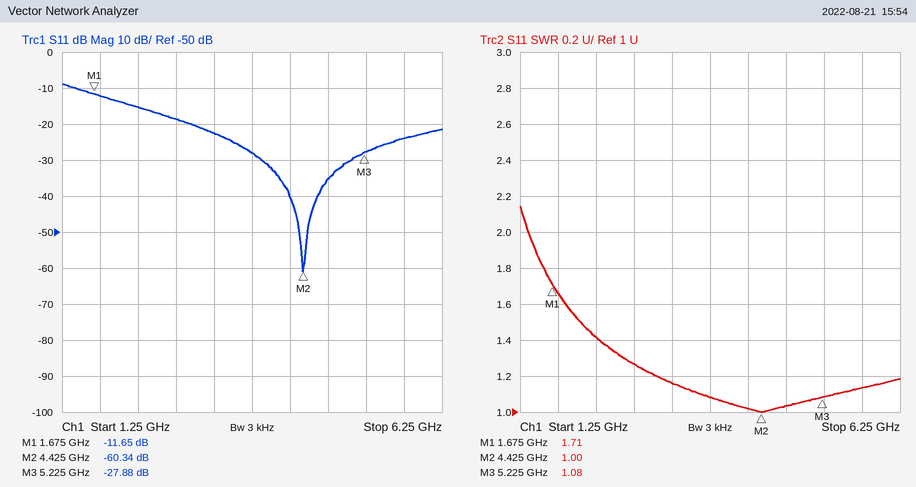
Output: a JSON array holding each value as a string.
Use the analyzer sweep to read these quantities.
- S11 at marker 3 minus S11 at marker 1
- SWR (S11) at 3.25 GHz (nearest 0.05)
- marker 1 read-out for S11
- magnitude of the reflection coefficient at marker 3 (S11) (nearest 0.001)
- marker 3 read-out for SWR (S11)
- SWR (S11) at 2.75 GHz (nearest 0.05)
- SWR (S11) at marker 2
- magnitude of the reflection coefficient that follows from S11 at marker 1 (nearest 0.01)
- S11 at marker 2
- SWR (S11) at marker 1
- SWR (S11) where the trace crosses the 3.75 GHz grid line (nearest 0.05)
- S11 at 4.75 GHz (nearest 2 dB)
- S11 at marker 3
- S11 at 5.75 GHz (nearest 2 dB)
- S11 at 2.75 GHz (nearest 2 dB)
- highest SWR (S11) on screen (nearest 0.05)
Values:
["-16.23 dB", "1.15", "-11.65 dB", "0.040", "1.08", "1.25", "1.00", "0.26", "-60.34 dB", "1.71", "1.10", "-36 dB", "-27.88 dB", "-24 dB", "-18 dB", "2.15"]
